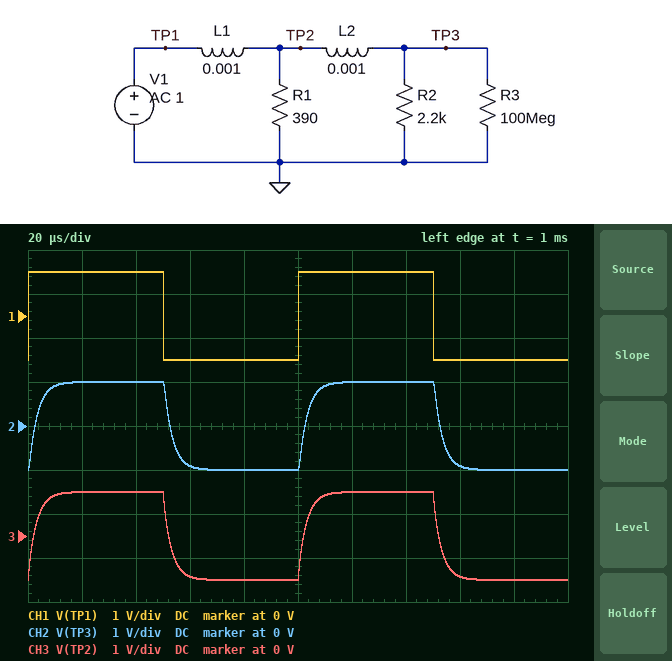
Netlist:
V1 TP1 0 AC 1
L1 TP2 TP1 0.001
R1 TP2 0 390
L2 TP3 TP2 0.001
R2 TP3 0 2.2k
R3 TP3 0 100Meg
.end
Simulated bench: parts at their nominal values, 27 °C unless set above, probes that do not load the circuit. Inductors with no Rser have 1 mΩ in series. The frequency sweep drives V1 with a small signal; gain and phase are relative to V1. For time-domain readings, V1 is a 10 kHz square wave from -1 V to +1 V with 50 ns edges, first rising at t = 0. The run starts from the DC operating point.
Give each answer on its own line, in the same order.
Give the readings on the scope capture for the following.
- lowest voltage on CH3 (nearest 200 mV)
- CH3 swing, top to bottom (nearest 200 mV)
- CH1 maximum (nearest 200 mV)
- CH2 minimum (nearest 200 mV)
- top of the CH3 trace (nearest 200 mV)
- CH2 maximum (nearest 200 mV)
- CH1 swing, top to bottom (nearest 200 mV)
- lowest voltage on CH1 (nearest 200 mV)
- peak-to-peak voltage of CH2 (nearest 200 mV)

-1.0 V
2.0 V
1.0 V
-1.0 V
1.0 V
1.0 V
2.0 V
-1.0 V
2.0 V
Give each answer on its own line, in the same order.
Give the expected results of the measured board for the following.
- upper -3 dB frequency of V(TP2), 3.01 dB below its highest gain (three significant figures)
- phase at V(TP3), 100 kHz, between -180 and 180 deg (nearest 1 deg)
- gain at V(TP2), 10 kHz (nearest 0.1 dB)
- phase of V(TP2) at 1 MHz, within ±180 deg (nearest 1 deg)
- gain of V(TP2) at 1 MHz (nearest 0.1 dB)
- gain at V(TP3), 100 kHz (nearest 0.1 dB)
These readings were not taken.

51.7 kHz
-76 deg
-0.2 dB
-83 deg
-24.4 dB
-7.0 dB
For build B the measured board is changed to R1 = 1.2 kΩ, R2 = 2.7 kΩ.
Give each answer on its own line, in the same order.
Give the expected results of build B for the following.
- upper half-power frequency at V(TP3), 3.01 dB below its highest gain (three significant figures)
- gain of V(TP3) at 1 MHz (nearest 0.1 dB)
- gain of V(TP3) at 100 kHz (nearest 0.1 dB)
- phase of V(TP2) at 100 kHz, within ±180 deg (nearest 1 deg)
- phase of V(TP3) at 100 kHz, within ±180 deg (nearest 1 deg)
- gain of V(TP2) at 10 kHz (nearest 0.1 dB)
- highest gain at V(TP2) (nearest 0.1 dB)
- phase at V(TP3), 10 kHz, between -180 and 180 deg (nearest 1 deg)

115 kHz
-23.5 dB
-2.4 dB
-35 deg
-48 deg
0 dB
0 dB
-6 deg
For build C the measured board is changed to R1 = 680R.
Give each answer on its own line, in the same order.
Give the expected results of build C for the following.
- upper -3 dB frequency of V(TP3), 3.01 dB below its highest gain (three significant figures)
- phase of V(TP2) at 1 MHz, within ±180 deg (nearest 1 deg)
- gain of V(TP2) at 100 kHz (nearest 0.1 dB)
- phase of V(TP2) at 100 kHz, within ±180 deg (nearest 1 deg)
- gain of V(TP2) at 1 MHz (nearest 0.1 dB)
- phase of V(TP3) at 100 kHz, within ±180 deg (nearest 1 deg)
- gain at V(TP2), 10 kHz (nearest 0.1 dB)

75.6 kHz
-79 deg
-4.1 dB
-48 deg
-19.8 dB
-64 deg
-0.1 dB
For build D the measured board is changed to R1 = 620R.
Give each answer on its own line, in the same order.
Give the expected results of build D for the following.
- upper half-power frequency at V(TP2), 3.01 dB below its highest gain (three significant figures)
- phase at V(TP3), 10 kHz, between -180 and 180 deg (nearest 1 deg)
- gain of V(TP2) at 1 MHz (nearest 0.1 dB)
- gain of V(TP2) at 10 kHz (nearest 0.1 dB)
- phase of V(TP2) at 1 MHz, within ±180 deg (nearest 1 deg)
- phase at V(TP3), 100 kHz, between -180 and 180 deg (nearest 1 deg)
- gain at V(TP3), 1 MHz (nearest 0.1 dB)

74.2 kHz
-9 deg
-20.5 dB
-0.1 dB
-80 deg
-66 deg
-30.1 dB
